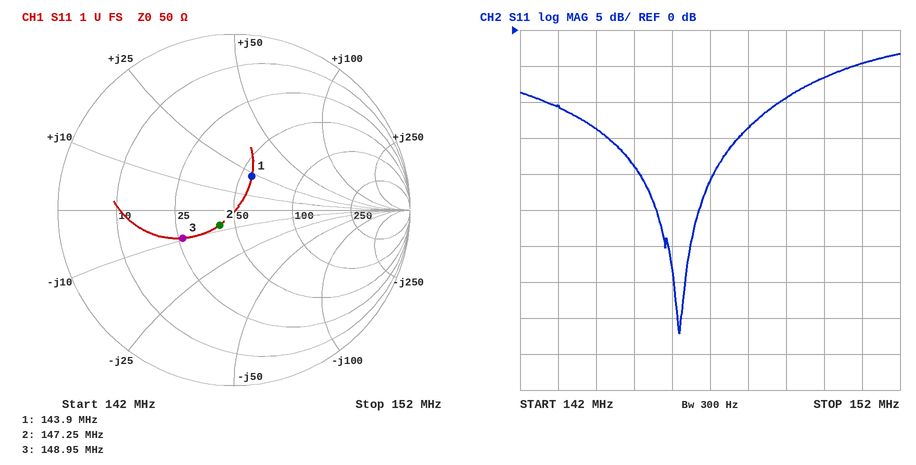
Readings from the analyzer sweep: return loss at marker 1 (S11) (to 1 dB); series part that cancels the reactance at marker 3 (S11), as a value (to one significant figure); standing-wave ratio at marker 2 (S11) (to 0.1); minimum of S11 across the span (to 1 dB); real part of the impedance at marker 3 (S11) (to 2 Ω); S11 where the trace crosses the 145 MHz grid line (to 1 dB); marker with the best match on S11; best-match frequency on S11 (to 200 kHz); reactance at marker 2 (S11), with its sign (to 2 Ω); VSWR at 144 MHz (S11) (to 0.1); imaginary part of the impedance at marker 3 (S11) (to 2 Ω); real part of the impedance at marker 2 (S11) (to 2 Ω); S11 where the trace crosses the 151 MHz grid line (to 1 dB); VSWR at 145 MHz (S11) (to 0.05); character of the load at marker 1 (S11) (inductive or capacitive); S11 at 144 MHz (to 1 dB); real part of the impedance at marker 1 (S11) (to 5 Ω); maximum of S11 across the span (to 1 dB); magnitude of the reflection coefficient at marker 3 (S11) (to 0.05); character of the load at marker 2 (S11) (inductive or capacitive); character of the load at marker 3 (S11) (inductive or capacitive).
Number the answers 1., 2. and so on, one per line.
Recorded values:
1. 13 dB
2. 10 nH
3. 1.3
4. -42 dB
5. 26 Ω
6. -19 dB
7. marker 2
8. 146.2 MHz
9. -8 Ω
10. 1.5
11. -10 Ω
12. 42 Ω
13. -5 dB
14. 1.25
15. inductive
16. -14 dB
17. 55 Ω
18. -3 dB
19. 0.35
20. capacitive
21. capacitive
